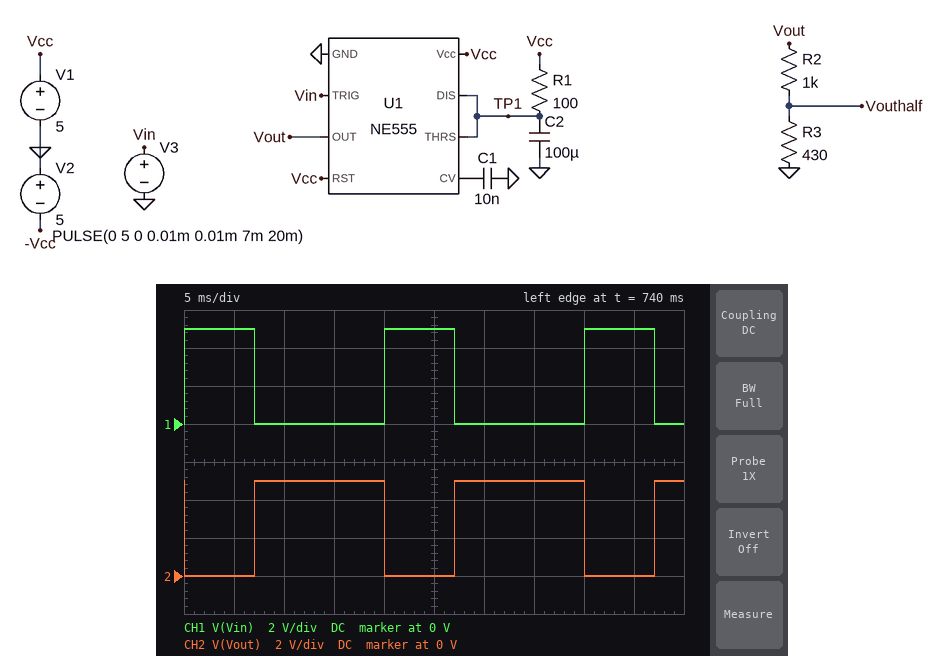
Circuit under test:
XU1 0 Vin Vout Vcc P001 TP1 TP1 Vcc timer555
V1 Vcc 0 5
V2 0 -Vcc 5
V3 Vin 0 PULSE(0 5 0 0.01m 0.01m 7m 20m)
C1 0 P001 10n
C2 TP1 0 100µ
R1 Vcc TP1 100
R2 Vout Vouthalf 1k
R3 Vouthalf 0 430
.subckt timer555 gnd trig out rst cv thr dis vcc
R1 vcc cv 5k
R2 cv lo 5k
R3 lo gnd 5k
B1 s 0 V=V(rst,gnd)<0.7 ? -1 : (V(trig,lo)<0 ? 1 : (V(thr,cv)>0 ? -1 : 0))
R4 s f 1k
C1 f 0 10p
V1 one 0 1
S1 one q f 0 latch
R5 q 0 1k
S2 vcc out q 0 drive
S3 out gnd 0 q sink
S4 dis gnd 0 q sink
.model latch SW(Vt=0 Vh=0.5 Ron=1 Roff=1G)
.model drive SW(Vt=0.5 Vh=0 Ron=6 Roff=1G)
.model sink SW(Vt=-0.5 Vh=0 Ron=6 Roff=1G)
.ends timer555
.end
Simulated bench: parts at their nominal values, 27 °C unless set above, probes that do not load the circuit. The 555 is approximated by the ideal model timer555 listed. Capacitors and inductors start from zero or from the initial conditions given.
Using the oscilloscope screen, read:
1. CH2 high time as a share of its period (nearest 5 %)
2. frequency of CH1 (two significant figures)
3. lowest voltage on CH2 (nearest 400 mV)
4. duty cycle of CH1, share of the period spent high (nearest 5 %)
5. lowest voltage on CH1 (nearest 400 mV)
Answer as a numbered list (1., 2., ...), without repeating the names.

1. 65 %
2. 50 Hz
3. 0 V
4. 35 %
5. 0 V
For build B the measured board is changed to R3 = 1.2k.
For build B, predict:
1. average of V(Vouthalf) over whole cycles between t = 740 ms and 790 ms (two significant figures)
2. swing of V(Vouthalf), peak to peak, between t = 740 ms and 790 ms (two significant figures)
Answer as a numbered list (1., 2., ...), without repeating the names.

1. 1.8 V
2. 2.7 V
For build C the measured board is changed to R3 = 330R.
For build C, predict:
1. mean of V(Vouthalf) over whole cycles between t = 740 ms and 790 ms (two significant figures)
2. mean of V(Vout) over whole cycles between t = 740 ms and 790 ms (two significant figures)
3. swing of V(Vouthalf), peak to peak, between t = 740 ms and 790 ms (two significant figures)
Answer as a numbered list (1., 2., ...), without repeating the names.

1. 800 mV
2. 3.2 V
3. 1.2 V
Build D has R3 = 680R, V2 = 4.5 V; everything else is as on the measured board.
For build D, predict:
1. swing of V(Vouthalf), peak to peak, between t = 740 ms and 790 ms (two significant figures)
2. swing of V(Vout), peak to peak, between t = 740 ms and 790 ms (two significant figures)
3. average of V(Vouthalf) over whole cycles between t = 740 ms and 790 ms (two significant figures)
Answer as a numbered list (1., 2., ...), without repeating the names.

1. 2.0 V
2. 5.0 V
3. 1.3 V
